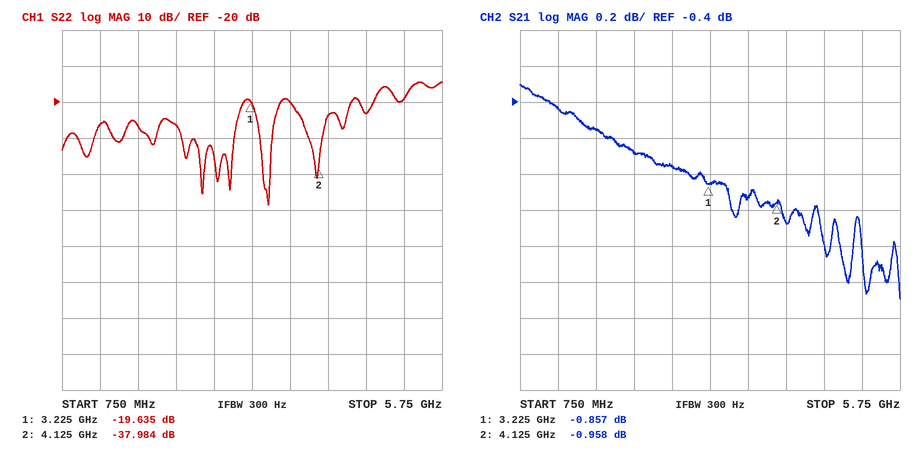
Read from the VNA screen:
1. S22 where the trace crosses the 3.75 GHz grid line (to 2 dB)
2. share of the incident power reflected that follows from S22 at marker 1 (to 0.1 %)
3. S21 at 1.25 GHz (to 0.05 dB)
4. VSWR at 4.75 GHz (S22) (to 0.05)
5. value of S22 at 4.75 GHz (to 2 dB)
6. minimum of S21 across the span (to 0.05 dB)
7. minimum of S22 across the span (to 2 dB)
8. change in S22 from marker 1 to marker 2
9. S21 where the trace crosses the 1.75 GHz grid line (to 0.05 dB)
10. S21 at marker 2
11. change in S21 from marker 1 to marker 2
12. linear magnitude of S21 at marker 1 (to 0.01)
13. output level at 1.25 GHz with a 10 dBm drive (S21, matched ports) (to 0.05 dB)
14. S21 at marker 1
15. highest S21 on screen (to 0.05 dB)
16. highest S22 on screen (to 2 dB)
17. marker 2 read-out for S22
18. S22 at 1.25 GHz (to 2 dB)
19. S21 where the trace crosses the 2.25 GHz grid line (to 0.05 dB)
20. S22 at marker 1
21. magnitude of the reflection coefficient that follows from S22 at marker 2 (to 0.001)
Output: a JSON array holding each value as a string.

["-20 dB", "1.1 %", "-0.45 dB", "1.15", "-24 dB", "-1.50 dB", "-48 dB", "-18.349 dB", "-0.55 dB", "-0.958 dB", "-0.101 dB", "0.91", "9.55 dBm", "-0.857 dB", "-0.30 dB", "-14 dB", "-37.984 dB", "-26 dB", "-0.70 dB", "-19.635 dB", "0.013"]
